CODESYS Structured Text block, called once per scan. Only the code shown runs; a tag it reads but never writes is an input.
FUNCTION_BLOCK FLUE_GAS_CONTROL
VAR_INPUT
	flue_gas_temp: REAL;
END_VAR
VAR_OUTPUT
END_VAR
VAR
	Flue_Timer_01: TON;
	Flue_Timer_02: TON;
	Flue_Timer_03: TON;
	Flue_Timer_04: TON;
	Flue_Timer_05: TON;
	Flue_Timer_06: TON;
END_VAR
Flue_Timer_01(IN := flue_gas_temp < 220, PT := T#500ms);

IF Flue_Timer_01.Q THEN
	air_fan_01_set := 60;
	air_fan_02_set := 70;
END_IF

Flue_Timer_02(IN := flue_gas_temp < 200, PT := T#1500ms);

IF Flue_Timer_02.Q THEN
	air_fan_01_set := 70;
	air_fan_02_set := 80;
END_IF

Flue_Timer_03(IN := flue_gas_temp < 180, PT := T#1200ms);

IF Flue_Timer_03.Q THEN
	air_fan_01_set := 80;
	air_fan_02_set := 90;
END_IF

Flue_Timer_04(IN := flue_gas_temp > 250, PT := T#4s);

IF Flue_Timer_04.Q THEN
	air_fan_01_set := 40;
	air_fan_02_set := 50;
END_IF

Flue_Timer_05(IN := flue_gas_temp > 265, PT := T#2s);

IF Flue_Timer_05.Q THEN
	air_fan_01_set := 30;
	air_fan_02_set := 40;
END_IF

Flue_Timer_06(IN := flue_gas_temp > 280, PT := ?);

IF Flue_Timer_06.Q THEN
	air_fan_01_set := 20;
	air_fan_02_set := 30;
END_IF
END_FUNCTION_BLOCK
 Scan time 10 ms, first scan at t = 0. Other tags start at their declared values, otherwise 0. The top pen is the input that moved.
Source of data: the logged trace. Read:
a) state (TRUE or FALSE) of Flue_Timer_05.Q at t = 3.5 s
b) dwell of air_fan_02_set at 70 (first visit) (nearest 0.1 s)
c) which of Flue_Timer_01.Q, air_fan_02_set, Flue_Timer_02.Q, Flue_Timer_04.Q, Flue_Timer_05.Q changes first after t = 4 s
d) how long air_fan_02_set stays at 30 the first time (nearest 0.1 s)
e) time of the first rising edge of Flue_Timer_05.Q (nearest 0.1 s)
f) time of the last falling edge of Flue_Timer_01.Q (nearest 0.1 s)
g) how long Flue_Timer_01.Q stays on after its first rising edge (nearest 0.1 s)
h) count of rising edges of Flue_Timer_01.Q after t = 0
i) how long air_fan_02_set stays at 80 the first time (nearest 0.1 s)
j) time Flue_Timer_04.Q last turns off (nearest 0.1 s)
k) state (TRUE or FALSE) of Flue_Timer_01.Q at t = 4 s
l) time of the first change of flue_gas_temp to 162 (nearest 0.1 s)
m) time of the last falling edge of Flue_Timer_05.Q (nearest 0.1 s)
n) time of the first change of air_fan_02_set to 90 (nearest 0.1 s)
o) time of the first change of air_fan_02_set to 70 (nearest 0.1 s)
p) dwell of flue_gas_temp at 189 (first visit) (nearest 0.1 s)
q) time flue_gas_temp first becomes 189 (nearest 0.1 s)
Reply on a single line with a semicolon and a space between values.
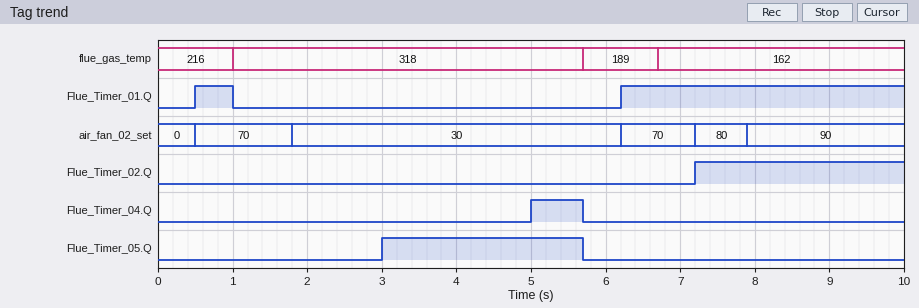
TRUE; 1.3 s; Flue_Timer_04.Q; 4.4 s; 3.0 s; 1.0 s; 0.5 s; 2; 0.7 s; 5.7 s; FALSE; 6.7 s; 5.7 s; 7.9 s; 0.5 s; 1.0 s; 5.7 s
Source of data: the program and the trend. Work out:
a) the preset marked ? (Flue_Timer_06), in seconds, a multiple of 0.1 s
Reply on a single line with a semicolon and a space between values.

0.8 s
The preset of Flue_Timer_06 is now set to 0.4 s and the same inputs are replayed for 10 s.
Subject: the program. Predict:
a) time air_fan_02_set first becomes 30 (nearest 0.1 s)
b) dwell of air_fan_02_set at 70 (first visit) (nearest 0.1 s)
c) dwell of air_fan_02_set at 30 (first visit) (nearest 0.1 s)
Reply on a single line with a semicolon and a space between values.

1.4 s; 0.9 s; 4.8 s
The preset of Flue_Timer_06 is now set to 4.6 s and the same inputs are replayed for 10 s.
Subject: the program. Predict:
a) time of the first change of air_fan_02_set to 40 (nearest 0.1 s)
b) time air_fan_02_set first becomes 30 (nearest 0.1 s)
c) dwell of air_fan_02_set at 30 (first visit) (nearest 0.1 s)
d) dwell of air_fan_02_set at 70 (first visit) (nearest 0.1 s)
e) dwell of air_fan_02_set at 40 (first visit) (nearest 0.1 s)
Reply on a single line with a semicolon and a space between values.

3.0 s; 5.6 s; 0.6 s; 2.5 s; 2.6 s
